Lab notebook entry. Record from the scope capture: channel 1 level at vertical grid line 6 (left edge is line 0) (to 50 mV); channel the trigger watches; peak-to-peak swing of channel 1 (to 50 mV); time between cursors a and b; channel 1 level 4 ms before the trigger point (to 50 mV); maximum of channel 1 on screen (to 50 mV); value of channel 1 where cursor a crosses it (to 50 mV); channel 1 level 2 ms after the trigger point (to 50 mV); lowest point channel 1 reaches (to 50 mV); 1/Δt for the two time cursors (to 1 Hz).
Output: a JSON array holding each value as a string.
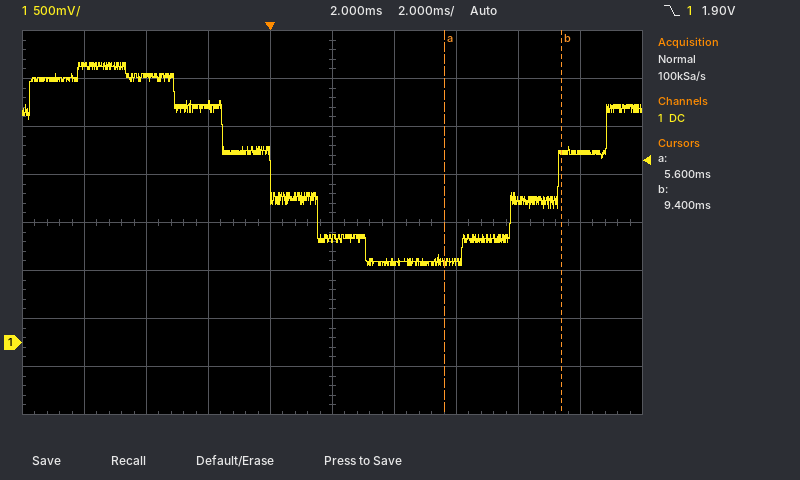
["850 mV", "channel 1", "2.10 V", "3.8 ms", "2.80 V", "2.90 V", "850 mV", "1.10 V", "800 mV", "263 Hz"]
